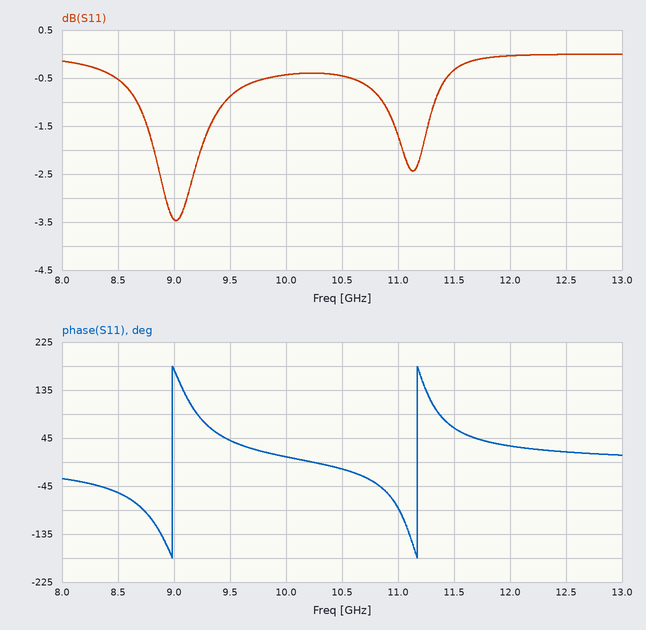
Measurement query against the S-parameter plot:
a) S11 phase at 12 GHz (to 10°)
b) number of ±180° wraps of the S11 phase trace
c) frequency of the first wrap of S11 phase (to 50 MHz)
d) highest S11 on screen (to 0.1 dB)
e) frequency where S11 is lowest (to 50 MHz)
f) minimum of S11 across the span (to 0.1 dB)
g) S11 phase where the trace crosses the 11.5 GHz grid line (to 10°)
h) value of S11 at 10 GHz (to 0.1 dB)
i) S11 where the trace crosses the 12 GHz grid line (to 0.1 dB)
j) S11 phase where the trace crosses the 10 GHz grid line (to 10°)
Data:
30°
2
9.00 GHz
0.0 dB
9.00 GHz
-3.5 dB
60°
-0.4 dB
0.0 dB
10°
